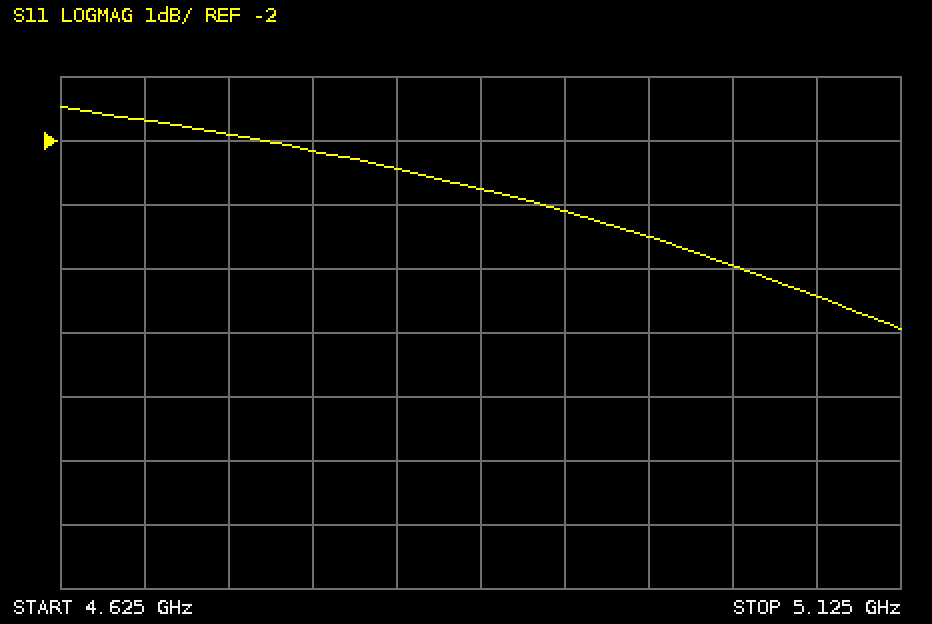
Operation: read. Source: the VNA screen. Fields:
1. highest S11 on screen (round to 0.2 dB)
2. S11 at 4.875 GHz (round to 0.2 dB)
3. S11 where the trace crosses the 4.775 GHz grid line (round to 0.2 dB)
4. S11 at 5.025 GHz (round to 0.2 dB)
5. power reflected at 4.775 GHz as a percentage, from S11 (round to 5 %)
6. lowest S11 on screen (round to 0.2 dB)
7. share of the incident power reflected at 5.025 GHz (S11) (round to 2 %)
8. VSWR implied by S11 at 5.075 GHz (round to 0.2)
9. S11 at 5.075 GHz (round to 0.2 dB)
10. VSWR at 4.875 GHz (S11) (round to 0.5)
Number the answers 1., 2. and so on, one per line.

1. -1.4 dB
2. -2.8 dB
3. -2.2 dB
4. -4.0 dB
5. 60 %
6. -5.0 dB
7. 40 %
8. 4.0
9. -4.4 dB
10. 6.5
